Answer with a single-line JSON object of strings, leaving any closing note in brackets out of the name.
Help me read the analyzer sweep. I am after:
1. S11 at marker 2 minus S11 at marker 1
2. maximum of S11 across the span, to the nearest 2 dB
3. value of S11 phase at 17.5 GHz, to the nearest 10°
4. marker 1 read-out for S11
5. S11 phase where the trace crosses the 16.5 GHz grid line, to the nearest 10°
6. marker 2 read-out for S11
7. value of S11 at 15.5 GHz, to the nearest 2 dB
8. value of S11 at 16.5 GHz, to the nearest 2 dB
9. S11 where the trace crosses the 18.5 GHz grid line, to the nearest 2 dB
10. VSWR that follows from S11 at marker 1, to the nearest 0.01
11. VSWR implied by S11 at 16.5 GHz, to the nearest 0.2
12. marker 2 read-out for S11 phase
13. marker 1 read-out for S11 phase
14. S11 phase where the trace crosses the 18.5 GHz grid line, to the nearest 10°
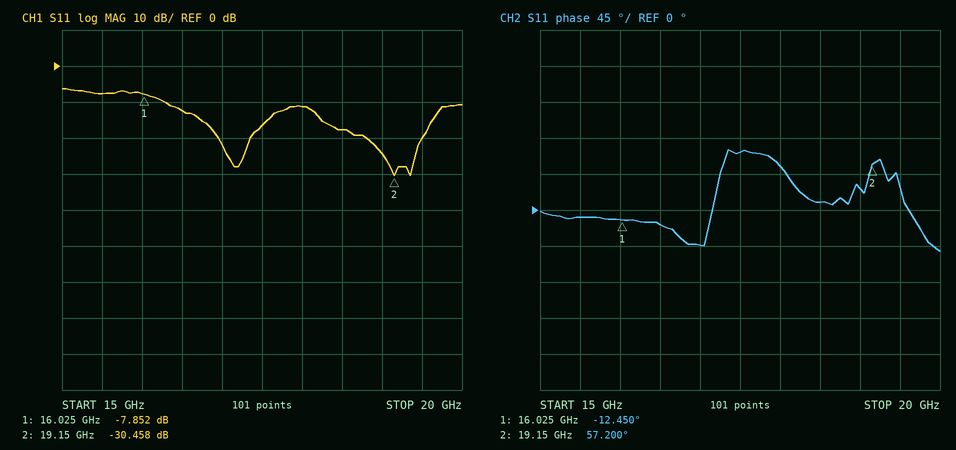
{"S11 at marker 2 minus S11 at marker 1": "-22.606 dB", "maximum of S11 across the span, to the nearest 2 dB": "-6 dB", "value of S11 phase at 17.5 GHz, to the nearest 10°": "70°", "marker 1 read-out for S11": "-7.852 dB", "S11 phase where the trace crosses the 16.5 GHz grid line, to the nearest 10°": "-20°", "marker 2 read-out for S11": "-30.458 dB", "value of S11 at 15.5 GHz, to the nearest 2 dB": "-8 dB", "value of S11 at 16.5 GHz, to the nearest 2 dB": "-12 dB", "S11 where the trace crosses the 18.5 GHz grid line, to the nearest 2 dB": "-18 dB", "VSWR that follows from S11 at marker 1, to the nearest 0.01": "2.36", "VSWR implied by S11 at 16.5 GHz, to the nearest 0.2": "1.6", "marker 2 read-out for S11 phase": "57.200°", "marker 1 read-out for S11 phase": "-12.450°", "S11 phase where the trace crosses the 18.5 GHz grid line, to the nearest 10°": "10°"}
